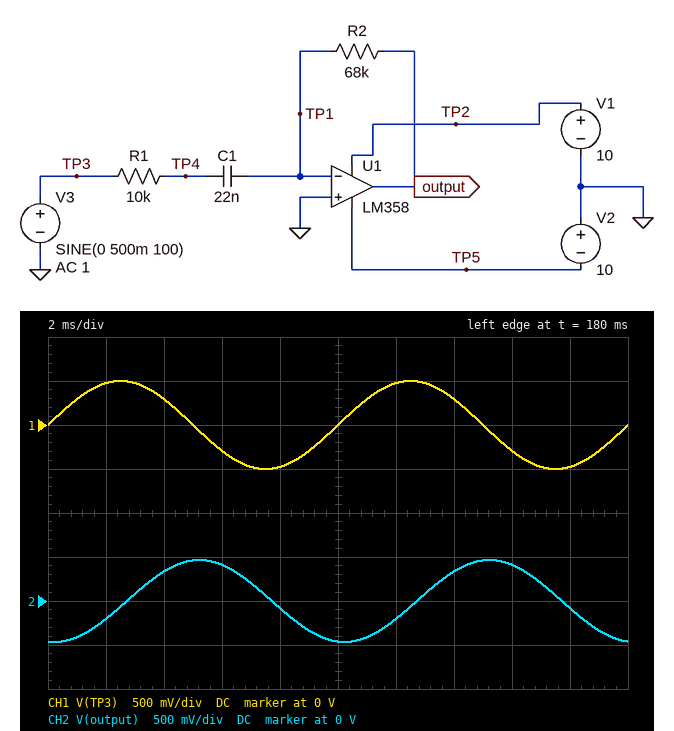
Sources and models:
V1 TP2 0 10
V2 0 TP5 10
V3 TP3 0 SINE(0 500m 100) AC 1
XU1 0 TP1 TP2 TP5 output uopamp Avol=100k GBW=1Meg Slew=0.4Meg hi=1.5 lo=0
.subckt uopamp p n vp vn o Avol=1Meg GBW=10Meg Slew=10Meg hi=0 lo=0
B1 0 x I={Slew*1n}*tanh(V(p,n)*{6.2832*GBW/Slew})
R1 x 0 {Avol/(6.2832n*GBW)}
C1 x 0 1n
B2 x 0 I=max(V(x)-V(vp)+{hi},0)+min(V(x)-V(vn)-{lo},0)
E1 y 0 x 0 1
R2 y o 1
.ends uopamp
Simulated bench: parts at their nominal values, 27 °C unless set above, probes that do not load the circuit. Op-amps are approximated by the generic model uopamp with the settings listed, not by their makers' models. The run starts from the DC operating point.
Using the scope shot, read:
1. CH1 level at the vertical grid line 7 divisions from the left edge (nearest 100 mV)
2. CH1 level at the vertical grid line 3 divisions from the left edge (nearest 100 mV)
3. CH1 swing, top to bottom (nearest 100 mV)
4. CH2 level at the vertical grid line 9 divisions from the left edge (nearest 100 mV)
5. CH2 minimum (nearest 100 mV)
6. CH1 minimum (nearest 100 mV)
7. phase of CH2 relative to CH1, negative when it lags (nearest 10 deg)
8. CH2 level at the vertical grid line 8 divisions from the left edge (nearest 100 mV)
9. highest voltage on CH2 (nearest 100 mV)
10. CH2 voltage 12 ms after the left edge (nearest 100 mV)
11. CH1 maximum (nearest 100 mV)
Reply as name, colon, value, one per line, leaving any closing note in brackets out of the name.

CH1 level at the vertical grid line 7 divisions from the left edge: 300 mV
CH1 level at the vertical grid line 3 divisions from the left edge: -300 mV
CH1 swing, top to bottom: 1.0 V
CH2 level at the vertical grid line 9 divisions from the left edge: -100 mV
CH2 minimum: -500 mV
CH1 minimum: -500 mV
phase of CH2 relative to CH1, negative when it lags: -100 deg
CH2 level at the vertical grid line 8 divisions from the left edge: 400 mV
highest voltage on CH2: 500 mV
CH2 voltage 12 ms after the left edge: -200 mV
CH1 maximum: 500 mV
